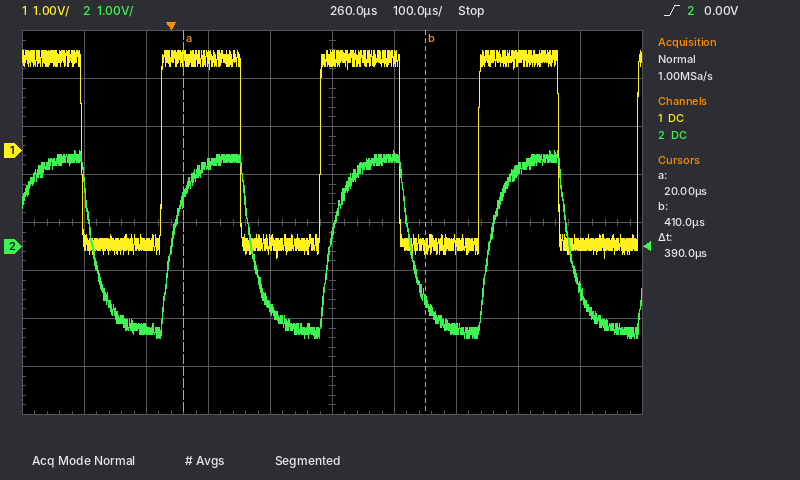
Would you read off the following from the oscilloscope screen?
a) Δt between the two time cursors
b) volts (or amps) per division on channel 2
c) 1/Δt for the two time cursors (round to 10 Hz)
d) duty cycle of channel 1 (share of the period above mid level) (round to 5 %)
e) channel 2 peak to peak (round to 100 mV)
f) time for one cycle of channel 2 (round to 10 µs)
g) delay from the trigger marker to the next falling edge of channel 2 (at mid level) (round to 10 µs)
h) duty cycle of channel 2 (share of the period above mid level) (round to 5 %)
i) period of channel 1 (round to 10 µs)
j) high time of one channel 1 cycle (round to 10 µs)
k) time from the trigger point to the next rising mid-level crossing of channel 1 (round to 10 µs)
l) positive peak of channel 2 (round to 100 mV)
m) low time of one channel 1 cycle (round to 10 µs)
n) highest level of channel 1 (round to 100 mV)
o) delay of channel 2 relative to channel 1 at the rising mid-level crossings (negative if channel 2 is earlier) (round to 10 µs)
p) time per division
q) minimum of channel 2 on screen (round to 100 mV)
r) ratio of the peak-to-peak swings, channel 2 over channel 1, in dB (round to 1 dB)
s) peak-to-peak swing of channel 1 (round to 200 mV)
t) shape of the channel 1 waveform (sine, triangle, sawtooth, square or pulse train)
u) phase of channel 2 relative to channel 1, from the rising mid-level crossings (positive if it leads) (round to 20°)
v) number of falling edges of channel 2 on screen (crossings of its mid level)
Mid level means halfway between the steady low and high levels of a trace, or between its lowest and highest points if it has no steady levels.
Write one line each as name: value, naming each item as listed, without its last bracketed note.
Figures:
Δt between the two time cursors: 390 µs
volts (or amps) per division on channel 2: 1 V
1/Δt for the two time cursors: 2.56 kHz
duty cycle of channel 1 (share of the period above mid level): 50 %
channel 2 peak to peak: 3.9 V
time for one cycle of channel 2: 260 µs
delay from the trigger marker to the next falling edge of channel 2 (at mid level): 130 µs
duty cycle of channel 2 (share of the period above mid level): 50 %
period of channel 1: 260 µs
high time of one channel 1 cycle: 130 µs
time from the trigger point to the next rising mid-level crossing of channel 1: 240 µs
positive peak of channel 2: 2.0 V
low time of one channel 1 cycle: 130 µs
highest level of channel 1: 2.1 V
delay of channel 2 relative to channel 1 at the rising mid-level crossings (negative if channel 2 is earlier): +20 µs
time per division: 100 µs
minimum of channel 2 on screen: -1.9 V
ratio of the peak-to-peak swings, channel 2 over channel 1, in dB: -1 dB
peak-to-peak swing of channel 1: 4.4 V
shape of the channel 1 waveform: square
phase of channel 2 relative to channel 1, from the rising mid-level crossings (positive if it leads): -20°
number of falling edges of channel 2 on screen: 4
